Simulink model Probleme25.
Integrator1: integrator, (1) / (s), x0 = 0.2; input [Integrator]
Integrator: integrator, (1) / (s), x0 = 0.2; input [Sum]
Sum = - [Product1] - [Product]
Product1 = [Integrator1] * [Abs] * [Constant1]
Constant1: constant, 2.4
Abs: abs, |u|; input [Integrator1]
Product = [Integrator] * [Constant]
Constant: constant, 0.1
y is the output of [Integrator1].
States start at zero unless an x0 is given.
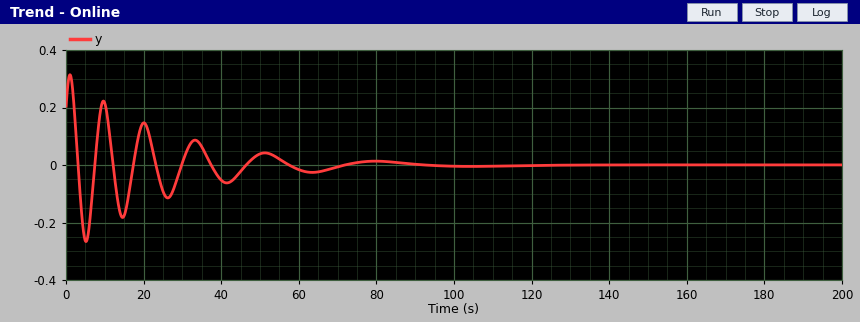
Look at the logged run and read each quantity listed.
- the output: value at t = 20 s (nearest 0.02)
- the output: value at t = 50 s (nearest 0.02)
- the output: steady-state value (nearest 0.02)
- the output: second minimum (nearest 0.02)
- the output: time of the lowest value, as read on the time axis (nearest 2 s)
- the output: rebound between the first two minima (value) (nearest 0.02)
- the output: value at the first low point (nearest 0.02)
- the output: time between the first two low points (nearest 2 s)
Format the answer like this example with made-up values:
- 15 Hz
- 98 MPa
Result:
- 0.14
- 0.04
- 0.00
- -0.18
- 6 s
- 0.22
- -0.26
- 10 s
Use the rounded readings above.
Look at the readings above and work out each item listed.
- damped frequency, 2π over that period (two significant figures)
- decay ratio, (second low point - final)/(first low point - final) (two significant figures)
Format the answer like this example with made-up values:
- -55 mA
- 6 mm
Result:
- 0.63 rad/s
- 0.69
